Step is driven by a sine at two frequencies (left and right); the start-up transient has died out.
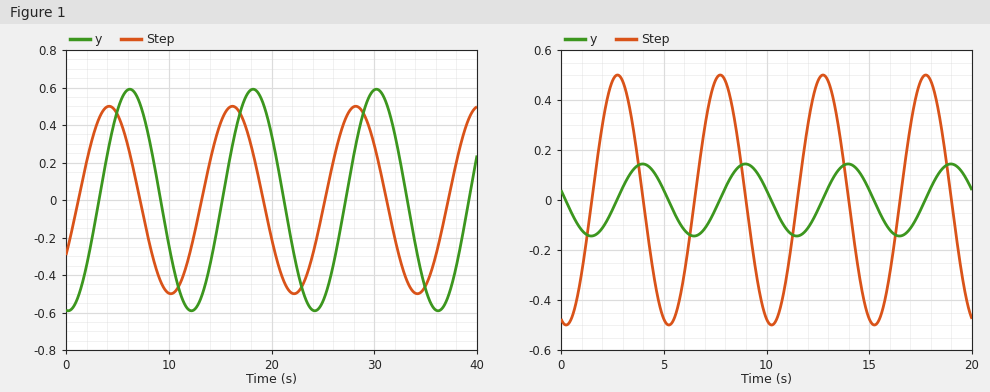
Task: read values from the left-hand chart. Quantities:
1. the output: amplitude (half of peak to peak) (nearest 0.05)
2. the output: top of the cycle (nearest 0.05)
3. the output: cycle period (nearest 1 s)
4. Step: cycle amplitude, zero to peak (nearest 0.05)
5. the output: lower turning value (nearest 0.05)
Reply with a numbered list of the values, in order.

1. 0.60
2. 0.60
3. 12 s
4. 0.50
5. -0.60
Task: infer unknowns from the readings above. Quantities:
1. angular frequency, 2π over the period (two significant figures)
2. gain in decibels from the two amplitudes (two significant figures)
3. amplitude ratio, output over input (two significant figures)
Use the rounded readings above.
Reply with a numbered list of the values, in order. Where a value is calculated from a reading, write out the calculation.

1. 2π / 12 = 0.52 rad/s
2. 20 log10(0.6 / 0.5) = 1.6 dB
3. 0.6 / 0.5 = 1.2
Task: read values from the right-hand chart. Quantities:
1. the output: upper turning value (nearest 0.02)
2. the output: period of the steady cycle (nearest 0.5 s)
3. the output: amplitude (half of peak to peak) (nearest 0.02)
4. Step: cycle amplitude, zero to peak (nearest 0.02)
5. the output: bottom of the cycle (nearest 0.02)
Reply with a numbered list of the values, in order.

1. 0.14
2. 5.0 s
3. 0.14
4. 0.50
5. -0.14
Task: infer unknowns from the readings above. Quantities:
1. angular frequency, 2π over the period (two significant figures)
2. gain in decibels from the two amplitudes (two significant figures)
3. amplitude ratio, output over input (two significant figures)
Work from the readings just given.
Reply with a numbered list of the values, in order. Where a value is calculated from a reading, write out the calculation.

1. 2π / 5 = 1.3 rad/s
2. 20 log10(0.14 / 0.5) = -11 dB
3. 0.14 / 0.5 = 0.28
